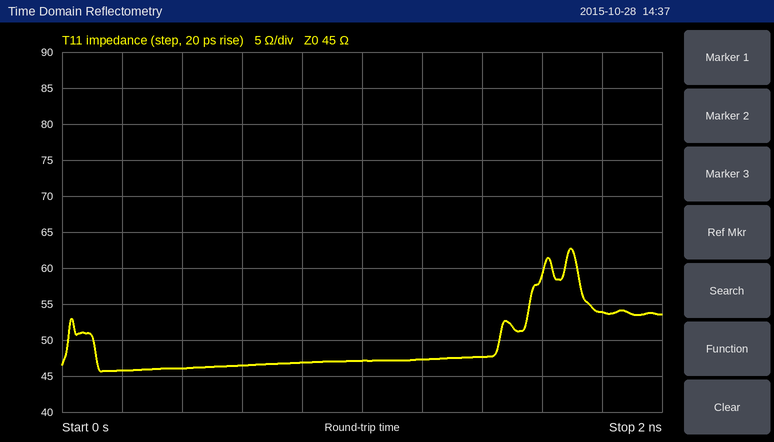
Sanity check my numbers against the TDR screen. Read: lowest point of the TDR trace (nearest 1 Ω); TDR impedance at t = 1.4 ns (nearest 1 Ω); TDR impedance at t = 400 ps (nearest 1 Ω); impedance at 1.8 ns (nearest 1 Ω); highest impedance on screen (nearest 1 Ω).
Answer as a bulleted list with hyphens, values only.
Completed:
- 46 Ω
- 48 Ω
- 46 Ω
- 54 Ω
- 63 Ω
